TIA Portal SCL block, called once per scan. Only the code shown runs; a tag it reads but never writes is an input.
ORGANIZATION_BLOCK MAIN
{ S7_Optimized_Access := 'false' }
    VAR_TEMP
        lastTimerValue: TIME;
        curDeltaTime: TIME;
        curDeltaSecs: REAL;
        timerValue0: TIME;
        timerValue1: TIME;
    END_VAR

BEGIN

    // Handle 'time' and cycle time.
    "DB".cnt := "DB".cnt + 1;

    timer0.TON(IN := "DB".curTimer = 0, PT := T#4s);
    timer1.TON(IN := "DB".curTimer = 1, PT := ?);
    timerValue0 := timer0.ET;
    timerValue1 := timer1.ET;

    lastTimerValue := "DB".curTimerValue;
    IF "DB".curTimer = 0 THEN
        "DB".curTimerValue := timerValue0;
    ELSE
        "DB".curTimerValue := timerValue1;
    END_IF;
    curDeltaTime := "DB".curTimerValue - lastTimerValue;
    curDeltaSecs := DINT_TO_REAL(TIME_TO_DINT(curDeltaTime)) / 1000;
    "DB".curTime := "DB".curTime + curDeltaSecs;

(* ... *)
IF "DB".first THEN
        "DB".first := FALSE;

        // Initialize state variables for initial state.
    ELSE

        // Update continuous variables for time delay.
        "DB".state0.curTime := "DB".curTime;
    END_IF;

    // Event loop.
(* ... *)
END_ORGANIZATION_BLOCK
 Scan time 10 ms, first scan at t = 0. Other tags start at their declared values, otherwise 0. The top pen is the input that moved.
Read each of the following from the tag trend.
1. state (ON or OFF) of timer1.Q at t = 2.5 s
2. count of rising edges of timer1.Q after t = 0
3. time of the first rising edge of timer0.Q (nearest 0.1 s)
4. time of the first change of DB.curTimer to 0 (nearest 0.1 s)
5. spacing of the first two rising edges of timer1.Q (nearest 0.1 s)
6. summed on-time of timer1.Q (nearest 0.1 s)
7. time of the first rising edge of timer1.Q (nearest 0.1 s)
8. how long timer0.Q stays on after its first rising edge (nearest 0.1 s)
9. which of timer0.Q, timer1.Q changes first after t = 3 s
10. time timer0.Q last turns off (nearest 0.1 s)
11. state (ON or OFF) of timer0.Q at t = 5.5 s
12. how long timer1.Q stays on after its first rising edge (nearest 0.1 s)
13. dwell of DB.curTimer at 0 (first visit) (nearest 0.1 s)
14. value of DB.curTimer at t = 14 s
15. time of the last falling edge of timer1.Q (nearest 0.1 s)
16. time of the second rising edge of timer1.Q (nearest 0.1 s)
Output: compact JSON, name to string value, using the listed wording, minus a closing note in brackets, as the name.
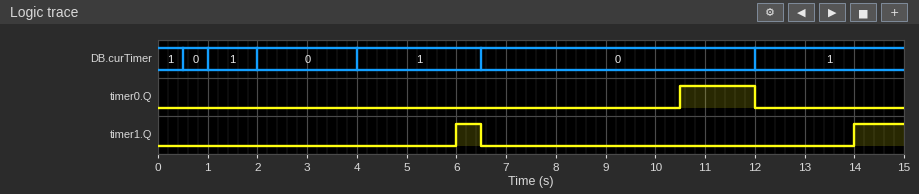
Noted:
{"state (ON or OFF) of timer1.Q at t = 2.5 s": "OFF", "count of rising edges of timer1.Q after t = 0": "2", "time of the first rising edge of timer0.Q": "10.5 s", "time of the first change of DB.curTimer to 0": "0.5 s", "spacing of the first two rising edges of timer1.Q": "8.0 s", "summed on-time of timer1.Q": "1.5 s", "time of the first rising edge of timer1.Q": "6.0 s", "how long timer0.Q stays on after its first rising edge": "1.5 s", "which of timer0.Q, timer1.Q changes first after t = 3 s": "timer1.Q", "time timer0.Q last turns off": "12.0 s", "state (ON or OFF) of timer0.Q at t = 5.5 s": "OFF", "how long timer1.Q stays on after its first rising edge": "0.5 s", "dwell of DB.curTimer at 0 (first visit)": "0.5 s", "value of DB.curTimer at t = 14 s": "1", "time of the last falling edge of timer1.Q": "6.5 s", "time of the second rising edge of timer1.Q": "14.0 s"}
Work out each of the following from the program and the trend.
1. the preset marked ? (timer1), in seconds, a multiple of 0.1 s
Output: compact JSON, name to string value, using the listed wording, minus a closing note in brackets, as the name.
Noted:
{"the preset marked ? (timer1), in seconds, a multiple of 0.1 s": "2.0 s"}
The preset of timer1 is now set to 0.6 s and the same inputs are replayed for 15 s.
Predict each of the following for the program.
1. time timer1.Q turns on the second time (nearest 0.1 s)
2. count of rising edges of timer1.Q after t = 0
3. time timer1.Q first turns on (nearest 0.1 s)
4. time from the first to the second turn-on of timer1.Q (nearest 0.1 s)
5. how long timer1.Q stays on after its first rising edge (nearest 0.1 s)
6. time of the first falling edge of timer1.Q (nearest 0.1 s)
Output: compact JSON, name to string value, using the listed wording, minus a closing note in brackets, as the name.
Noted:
{"time timer1.Q turns on the second time": "4.6 s", "count of rising edges of timer1.Q after t = 0": "3", "time timer1.Q first turns on": "1.6 s", "time from the first to the second turn-on of timer1.Q": "3.0 s", "how long timer1.Q stays on after its first rising edge": "0.4 s", "time of the first falling edge of timer1.Q": "2.0 s"}
